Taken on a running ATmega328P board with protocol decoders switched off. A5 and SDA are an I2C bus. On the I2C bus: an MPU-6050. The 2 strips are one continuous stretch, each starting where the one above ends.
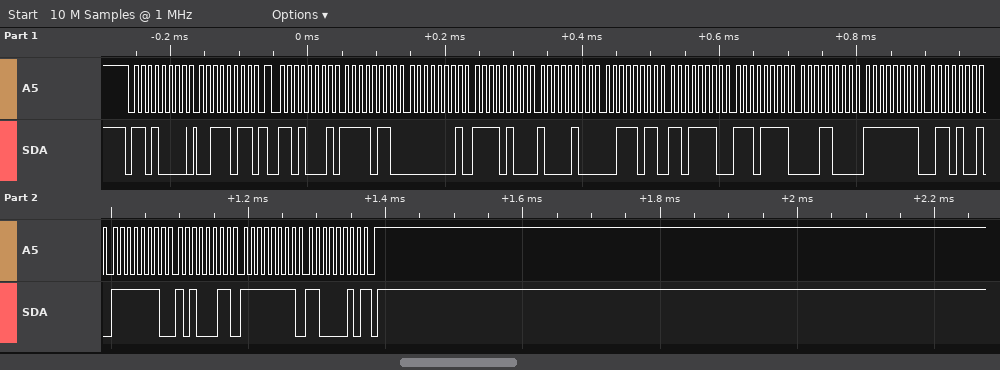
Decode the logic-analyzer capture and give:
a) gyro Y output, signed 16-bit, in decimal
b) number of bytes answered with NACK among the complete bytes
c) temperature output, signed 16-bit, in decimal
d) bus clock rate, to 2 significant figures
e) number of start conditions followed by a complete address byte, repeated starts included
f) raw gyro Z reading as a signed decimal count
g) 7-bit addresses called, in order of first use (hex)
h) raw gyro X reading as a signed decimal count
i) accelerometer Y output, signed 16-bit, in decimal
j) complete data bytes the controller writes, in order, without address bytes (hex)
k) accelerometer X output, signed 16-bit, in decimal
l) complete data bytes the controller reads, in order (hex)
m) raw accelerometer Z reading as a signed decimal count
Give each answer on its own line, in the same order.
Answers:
-349
1
-4328
100 kHz
2
-62
0x68
-151
-2940
3B
-2559
F6 01 F4 84 3B DE EF 18 FF 69 FE A3 FF C2
15326
